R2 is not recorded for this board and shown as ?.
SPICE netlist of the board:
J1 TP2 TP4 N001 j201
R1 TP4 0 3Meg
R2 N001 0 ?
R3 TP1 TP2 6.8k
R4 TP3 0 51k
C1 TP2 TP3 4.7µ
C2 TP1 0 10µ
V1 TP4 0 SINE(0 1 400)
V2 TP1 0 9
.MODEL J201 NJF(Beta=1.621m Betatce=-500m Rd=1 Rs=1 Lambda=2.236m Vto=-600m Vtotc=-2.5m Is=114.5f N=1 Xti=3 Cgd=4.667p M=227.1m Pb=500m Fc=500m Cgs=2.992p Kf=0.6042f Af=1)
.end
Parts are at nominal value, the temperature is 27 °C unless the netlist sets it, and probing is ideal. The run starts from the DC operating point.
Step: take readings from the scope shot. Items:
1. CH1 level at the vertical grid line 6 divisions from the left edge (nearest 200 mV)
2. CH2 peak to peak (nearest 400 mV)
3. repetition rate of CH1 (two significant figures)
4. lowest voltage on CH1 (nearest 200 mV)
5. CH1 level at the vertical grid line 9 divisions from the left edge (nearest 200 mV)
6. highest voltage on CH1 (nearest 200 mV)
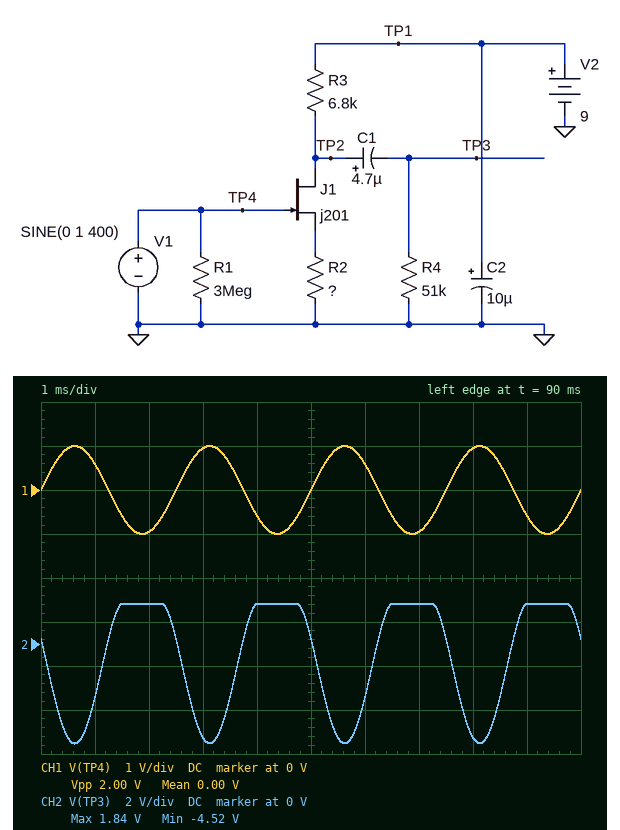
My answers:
600 mV
6.4 V
400 Hz
-1.0 V
-600 mV
1.0 V
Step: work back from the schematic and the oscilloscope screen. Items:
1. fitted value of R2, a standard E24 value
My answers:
750 Ω
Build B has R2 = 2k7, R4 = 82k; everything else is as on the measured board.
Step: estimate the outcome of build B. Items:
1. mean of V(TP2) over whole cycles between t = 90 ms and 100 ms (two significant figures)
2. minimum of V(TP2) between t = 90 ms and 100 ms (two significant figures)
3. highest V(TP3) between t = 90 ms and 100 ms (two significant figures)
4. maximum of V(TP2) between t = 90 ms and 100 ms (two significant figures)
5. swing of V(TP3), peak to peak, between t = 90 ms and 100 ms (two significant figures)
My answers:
7.9 V
6.4 V
820 mV
8.9 V
2.6 V
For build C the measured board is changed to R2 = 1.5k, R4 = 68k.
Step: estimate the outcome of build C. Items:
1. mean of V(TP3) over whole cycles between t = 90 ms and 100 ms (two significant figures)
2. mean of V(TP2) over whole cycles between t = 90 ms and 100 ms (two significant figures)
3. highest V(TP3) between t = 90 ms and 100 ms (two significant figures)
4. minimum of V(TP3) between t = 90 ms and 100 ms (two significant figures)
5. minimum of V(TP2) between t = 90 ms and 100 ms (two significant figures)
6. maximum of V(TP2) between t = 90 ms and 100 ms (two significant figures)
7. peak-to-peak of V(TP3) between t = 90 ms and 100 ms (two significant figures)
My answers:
-330 mV
7.3 V
1.2 V
-2.8 V
4.9 V
8.9 V
4.0 V
